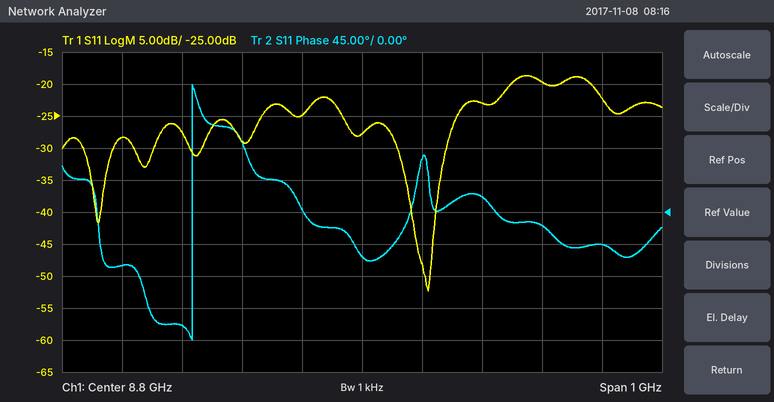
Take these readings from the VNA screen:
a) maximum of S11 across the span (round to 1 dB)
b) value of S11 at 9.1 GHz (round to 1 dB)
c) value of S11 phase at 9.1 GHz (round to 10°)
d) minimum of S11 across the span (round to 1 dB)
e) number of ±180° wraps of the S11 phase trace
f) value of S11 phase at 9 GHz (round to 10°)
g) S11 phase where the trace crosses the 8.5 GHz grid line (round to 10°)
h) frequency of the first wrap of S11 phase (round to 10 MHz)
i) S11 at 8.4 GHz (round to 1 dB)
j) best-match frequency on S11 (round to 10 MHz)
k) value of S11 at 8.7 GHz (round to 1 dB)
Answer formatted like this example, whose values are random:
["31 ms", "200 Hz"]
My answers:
["-19 dB", "-20 dB", "-20°", "-52 dB", "1", "20°", "-160°", "8.52 GHz", "-28 dB", "8.91 GHz", "-25 dB"]
